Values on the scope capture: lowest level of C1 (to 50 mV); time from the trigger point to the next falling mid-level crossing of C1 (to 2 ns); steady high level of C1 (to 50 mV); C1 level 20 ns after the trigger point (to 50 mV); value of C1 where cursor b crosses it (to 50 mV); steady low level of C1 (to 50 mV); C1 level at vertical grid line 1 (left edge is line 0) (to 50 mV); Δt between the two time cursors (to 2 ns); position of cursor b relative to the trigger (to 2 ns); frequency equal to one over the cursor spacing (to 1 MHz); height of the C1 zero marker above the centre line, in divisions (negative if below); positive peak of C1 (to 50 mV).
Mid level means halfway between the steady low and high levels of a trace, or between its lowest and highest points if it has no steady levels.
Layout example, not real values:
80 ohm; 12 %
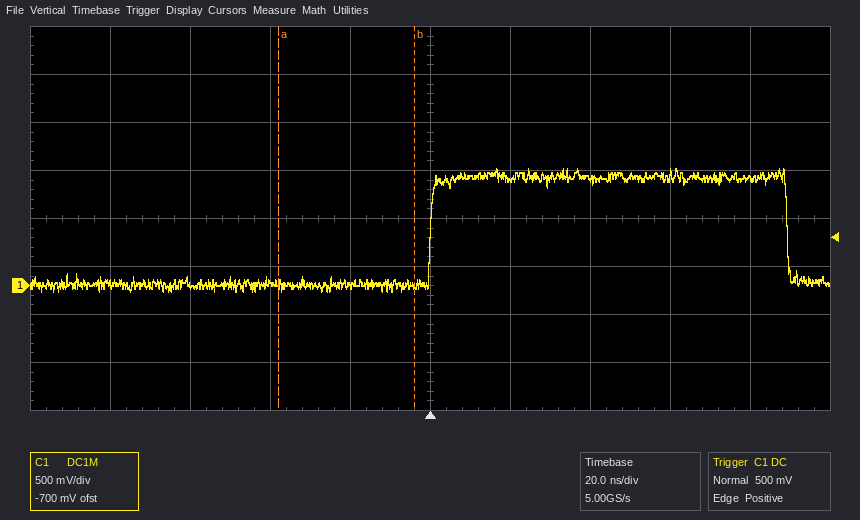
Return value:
-50 mV; 90 ns; 1.15 V; 1.10 V; 0 mV; 0 mV; 0 mV; 34 ns; -4 ns; 29 MHz; -1.4 div; 1.20 V
